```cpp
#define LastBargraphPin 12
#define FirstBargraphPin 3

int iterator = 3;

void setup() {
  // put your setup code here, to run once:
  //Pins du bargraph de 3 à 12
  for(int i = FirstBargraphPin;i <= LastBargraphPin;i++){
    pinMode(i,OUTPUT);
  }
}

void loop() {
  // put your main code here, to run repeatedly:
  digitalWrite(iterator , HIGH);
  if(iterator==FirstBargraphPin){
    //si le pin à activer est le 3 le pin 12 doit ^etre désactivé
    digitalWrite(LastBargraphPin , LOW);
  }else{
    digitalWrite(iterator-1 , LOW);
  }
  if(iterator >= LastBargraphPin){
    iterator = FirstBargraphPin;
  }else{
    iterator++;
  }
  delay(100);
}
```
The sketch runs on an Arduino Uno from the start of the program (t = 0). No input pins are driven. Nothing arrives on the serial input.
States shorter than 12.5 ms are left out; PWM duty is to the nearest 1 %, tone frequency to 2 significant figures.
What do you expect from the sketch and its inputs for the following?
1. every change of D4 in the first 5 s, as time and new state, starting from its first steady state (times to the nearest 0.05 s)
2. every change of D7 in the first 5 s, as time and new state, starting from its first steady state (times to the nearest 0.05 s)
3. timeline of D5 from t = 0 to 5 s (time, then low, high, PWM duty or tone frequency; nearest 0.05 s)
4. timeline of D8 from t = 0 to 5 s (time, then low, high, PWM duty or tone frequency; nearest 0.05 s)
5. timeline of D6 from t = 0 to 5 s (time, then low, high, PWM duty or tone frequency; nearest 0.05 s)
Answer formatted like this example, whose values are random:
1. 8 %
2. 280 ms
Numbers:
1. 0 s low; 0.1 s high; 0.2 s low; 1.1 s high; 1.2 s low; 2.1 s high; 2.2 s low; 3.1 s high; 3.2 s low; 4.1 s high; 4.2 s low
2. 0 s low; 0.4 s high; 0.5 s low; 1.4 s high; 1.5 s low; 2.4 s high; 2.5 s low; 3.4 s high; 3.5 s low; 4.4 s high; 4.5 s low
3. 0 s low; 0.2 s high; 0.3 s low; 1.2 s high; 1.3 s low; 2.2 s high; 2.3 s low; 3.2 s high; 3.3 s low; 4.2 s high; 4.3 s low
4. 0 s low; 0.5 s high; 0.6 s low; 1.5 s high; 1.6 s low; 2.5 s high; 2.6 s low; 3.5 s high; 3.6 s low; 4.5 s high; 4.6 s low
5. 0 s low; 0.3 s high; 0.4 s low; 1.3 s high; 1.4 s low; 2.3 s high; 2.4 s low; 3.3 s high; 3.4 s low; 4.3 s high; 4.4 s low
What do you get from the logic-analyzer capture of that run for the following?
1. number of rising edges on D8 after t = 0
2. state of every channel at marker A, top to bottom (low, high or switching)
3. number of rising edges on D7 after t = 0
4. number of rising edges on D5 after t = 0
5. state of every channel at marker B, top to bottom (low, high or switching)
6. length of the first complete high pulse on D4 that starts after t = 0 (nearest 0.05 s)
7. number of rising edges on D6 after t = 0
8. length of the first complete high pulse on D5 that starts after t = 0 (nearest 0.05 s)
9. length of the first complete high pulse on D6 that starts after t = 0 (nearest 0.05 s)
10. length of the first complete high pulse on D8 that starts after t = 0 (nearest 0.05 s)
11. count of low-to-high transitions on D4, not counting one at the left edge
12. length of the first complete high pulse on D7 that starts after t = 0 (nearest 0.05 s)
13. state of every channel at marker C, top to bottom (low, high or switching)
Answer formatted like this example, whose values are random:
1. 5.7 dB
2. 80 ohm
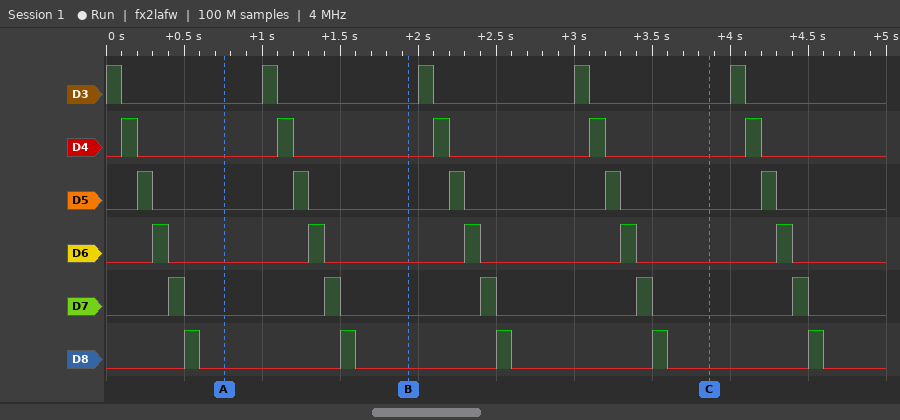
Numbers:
1. 5
2. D3 low, D4 low, D5 low, D6 low, D7 low, D8 low
3. 5
4. 5
5. D3 low, D4 low, D5 low, D6 low, D7 low, D8 low
6. 0.10 s
7. 5
8. 0.10 s
9. 0.10 s
10. 0.10 s
11. 5
12. 0.10 s
13. D3 low, D4 low, D5 low, D6 low, D7 low, D8 low
